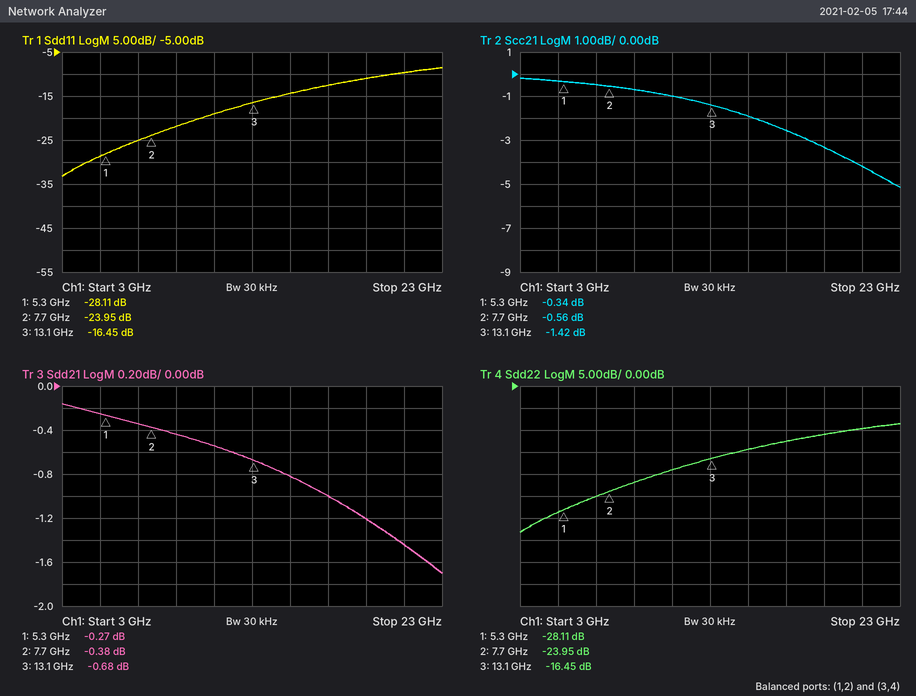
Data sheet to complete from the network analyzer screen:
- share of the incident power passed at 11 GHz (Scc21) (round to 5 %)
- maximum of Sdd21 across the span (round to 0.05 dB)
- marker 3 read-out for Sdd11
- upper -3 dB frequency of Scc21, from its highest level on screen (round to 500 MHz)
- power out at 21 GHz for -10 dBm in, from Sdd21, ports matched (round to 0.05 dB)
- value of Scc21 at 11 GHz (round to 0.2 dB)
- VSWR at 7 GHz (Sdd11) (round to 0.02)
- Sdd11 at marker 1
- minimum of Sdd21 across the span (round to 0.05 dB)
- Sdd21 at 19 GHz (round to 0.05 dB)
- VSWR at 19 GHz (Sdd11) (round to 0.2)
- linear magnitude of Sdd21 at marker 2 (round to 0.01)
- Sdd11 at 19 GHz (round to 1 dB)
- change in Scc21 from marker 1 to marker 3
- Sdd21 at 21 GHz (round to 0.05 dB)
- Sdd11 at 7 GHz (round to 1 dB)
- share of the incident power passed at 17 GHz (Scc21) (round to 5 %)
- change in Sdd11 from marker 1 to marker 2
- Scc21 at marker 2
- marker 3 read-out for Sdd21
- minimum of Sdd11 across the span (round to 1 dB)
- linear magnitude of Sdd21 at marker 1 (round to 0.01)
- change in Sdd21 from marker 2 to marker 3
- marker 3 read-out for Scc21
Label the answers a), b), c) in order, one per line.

a) 80 %
b) -0.15 dB
c) -16.45 dB
d) 18.5 GHz
e) -11.45 dBm
f) -1.0 dB
g) 1.12
h) -28.11 dB
i) -1.70 dB
j) -1.20 dB
k) 1.8
l) 0.96
m) -11 dB
n) -1.08 dB
o) -1.45 dB
p) -25 dB
q) 55 %
r) 4.16 dB
s) -0.56 dB
t) -0.68 dB
u) -33 dB
v) 0.97
w) -0.30 dB
x) -1.42 dB
